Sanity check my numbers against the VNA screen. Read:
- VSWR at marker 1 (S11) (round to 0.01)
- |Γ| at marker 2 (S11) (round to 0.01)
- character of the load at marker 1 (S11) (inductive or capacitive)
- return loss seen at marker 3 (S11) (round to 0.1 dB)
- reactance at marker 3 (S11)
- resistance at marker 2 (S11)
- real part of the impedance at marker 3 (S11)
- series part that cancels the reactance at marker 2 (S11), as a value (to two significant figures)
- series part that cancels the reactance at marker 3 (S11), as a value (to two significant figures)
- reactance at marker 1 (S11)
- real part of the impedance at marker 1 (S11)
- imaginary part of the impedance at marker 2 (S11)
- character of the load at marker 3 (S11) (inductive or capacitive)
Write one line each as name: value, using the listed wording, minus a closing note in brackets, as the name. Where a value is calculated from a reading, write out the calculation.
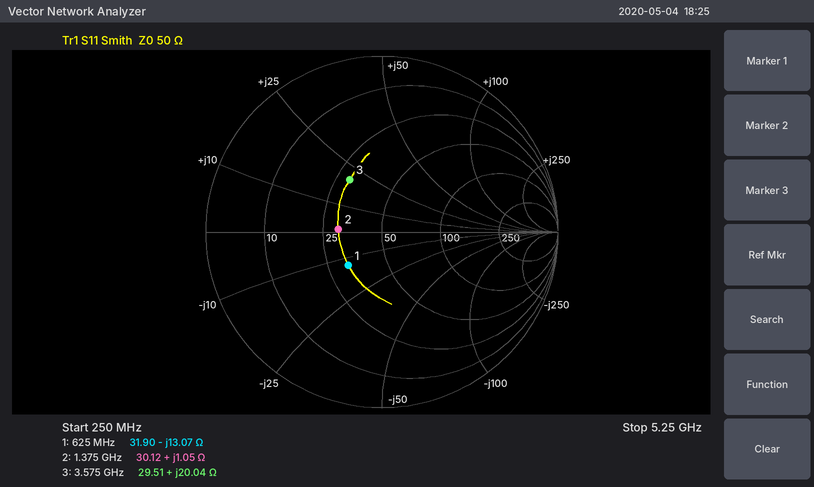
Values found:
VSWR at marker 1 (S11): 1.74
|Γ| at marker 2 (S11): 0.25
character of the load at marker 1 (S11): capacitive
return loss seen at marker 3 (S11): 9.1 dB
reactance at marker 3: +20.04 Ω
resistance at marker 2: 30.12 Ω
real part of the impedance at marker 3: 29.51 Ω
series part that cancels the reactance at marker 2 (S11), as a value: C = 1/(2π × 1.375 GHz × 1.05 Ω) ≈ 110 pF
series part that cancels the reactance at marker 3 (S11), as a value: C = 1/(2π × 3.575 GHz × 20.04 Ω) ≈ 2.2 pF
reactance at marker 1: -13.07 Ω
real part of the impedance at marker 1: 31.90 Ω
imaginary part of the impedance at marker 2: +1.05 Ω
character of the load at marker 3 (S11): inductive
